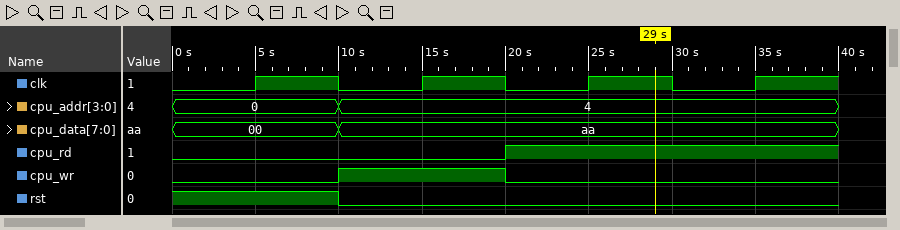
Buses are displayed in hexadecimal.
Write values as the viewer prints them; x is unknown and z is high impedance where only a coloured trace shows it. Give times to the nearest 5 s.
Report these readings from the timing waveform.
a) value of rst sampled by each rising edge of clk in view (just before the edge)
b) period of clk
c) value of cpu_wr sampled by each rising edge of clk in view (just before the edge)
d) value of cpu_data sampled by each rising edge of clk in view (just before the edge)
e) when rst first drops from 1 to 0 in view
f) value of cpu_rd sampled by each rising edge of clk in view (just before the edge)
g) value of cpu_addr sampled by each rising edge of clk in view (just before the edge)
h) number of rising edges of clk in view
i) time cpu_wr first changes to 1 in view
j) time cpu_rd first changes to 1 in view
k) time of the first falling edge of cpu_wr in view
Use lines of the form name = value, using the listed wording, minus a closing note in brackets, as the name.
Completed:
value of rst sampled by each rising edge of clk in view = 1 0 0 0
period of clk = 10 s
value of cpu_wr sampled by each rising edge of clk in view = 0 1 0 0
value of cpu_data sampled by each rising edge of clk in view = 00, aa, aa, aa
when rst first drops from 1 to 0 in view = 10 s
value of cpu_rd sampled by each rising edge of clk in view = 0 0 1 1
value of cpu_addr sampled by each rising edge of clk in view = 0, 4, 4, 4
number of rising edges of clk in view = 4
time cpu_wr first changes to 1 in view = 10 s
time cpu_rd first changes to 1 in view = 20 s
time of the first falling edge of cpu_wr in view = 20 s
